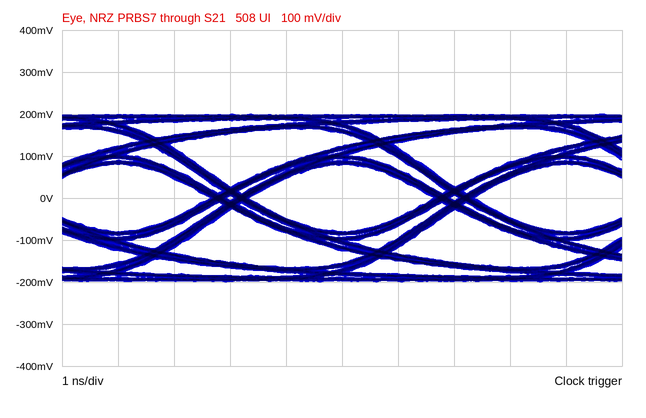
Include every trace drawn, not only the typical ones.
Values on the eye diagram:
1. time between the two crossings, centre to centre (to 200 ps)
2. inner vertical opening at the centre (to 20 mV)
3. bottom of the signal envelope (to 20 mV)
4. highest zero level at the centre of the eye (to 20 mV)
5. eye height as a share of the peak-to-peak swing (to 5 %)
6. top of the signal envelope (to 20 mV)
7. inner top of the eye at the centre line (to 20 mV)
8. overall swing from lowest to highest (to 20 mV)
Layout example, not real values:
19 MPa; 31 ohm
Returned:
4.0 ns; 160 mV; -200 mV; -80 mV; 40 %; 200 mV; 80 mV; 400 mV
